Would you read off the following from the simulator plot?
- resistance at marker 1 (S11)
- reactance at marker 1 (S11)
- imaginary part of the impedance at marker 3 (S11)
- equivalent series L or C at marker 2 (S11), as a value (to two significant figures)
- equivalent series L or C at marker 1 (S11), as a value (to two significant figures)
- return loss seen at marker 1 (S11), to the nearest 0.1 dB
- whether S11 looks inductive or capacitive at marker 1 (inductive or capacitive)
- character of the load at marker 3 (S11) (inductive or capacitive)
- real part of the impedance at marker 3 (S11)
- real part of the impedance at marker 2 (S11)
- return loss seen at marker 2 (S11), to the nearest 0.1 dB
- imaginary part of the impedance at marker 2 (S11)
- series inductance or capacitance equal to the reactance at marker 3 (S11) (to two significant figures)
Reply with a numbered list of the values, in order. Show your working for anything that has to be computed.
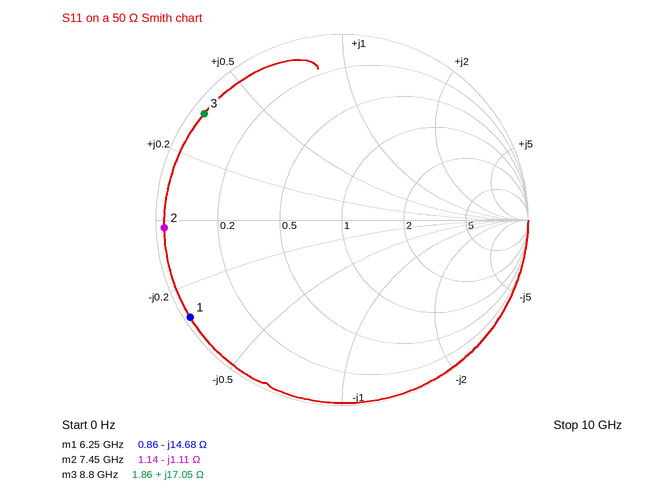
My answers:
1. 0.86 Ω
2. -14.68 Ω
3. +17.05 Ω
4. C = 1/(2π × 7.45 GHz × 1.11 Ω) ≈ 19 pF
5. C = 1/(2π × 6.25 GHz × 14.68 Ω) ≈ 1.7 pF
6. 0.3 dB
7. capacitive
8. inductive
9. 1.86 Ω
10. 1.14 Ω
11. 0.4 dB
12. -1.11 Ω
13. L = 17.05 Ω/(2π × 8.8 GHz) ≈ 308 pH, so 310 pH to two significant figures
